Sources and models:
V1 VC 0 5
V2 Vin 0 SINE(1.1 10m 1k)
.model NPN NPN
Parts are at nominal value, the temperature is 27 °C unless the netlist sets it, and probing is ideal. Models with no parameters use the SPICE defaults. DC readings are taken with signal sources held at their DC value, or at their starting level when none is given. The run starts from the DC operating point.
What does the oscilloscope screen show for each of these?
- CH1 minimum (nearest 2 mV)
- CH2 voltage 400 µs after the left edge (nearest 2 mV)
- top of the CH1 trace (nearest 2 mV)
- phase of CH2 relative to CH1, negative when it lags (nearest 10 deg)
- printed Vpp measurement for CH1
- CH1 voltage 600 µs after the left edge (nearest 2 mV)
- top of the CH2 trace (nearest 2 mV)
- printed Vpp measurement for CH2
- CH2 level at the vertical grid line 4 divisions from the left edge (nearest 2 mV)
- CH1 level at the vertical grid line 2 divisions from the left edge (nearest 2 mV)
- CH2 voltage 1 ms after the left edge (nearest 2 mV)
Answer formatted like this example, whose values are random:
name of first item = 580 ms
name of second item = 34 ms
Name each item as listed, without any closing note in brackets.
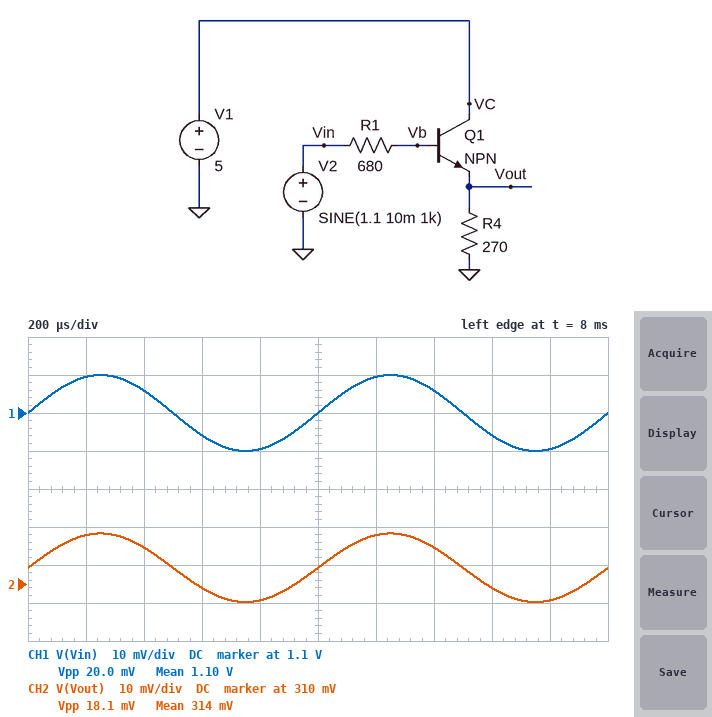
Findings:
CH1 minimum = 1.090 V
CH2 voltage 400 µs after the left edge = 320 mV
top of the CH1 trace = 1.110 V
phase of CH2 relative to CH1, negative when it lags = 0 deg
printed Vpp measurement for CH1 = 20.0 mV
CH1 voltage 600 µs after the left edge = 1.094 V
top of the CH2 trace = 324 mV
printed Vpp measurement for CH2 = 18.1 mV
CH2 level at the vertical grid line 4 divisions from the left edge = 306 mV
CH1 level at the vertical grid line 2 divisions from the left edge = 1.106 V
CH2 voltage 1 ms after the left edge = 314 mV
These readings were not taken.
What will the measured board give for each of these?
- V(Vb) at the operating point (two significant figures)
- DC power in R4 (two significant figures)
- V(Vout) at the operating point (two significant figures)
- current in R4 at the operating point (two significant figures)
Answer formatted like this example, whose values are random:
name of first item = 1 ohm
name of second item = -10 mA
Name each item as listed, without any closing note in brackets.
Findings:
V(Vb) at the operating point = 1.1 V
DC power in R4 = 370 µW
V(Vout) at the operating point = 310 mV
current in R4 at the operating point = 1.2 mA
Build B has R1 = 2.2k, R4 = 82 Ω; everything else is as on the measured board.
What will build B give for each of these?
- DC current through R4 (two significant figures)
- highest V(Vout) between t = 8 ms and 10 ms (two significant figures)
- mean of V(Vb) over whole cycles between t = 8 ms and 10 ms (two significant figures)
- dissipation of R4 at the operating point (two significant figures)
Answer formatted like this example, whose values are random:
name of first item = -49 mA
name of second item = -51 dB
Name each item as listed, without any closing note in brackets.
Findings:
DC current through R4 = 2.9 mA
highest V(Vout) between t = 8 ms and 10 ms = 240 mV
mean of V(Vb) over whole cycles between t = 8 ms and 10 ms = 1.0 V
dissipation of R4 at the operating point = 680 µW
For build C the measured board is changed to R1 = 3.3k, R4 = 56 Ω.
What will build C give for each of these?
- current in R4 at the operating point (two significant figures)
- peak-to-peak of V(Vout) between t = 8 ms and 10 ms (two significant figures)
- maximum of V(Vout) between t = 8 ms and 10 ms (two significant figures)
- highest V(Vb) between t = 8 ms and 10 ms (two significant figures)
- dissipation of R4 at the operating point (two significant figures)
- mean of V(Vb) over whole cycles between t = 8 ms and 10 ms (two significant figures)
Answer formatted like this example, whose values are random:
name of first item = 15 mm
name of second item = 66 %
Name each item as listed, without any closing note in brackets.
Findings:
current in R4 at the operating point = 3.3 mA
peak-to-peak of V(Vout) between t = 8 ms and 10 ms = 12 mV
maximum of V(Vout) between t = 8 ms and 10 ms = 190 mV
highest V(Vb) between t = 8 ms and 10 ms = 1.0 V
dissipation of R4 at the operating point = 620 µW
mean of V(Vb) over whole cycles between t = 8 ms and 10 ms = 990 mV
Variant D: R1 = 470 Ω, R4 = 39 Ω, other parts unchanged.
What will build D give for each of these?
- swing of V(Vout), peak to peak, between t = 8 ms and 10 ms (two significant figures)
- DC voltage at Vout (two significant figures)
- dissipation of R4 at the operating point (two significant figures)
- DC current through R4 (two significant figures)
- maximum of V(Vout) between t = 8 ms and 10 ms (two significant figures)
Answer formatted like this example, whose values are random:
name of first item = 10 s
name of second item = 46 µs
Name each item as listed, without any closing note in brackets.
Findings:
swing of V(Vout), peak to peak, between t = 8 ms and 10 ms = 16 mV
DC voltage at Vout = 250 mV
dissipation of R4 at the operating point = 1.6 mW
DC current through R4 = 6.4 mA
maximum of V(Vout) between t = 8 ms and 10 ms = 260 mV
